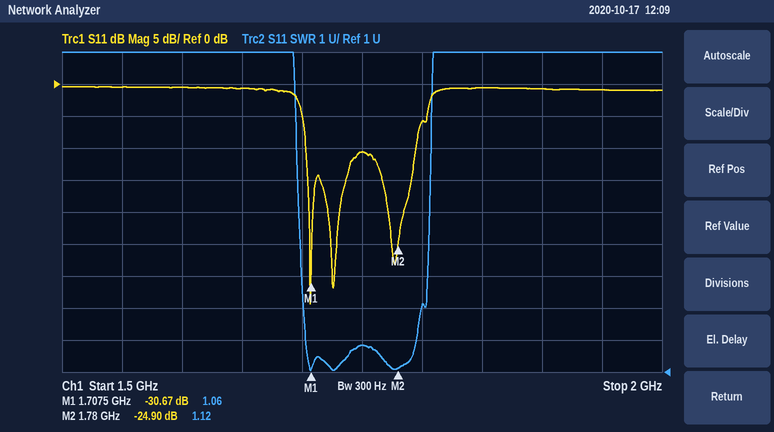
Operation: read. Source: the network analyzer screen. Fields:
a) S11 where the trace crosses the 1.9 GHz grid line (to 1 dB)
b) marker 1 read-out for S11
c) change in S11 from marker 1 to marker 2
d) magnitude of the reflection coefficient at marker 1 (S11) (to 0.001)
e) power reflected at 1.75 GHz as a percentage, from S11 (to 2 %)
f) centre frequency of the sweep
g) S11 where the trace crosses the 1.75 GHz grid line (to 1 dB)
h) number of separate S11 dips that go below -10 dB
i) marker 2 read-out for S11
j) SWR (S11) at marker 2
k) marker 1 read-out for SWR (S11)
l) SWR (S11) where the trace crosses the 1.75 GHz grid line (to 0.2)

-1 dB
-30.67 dB
5.77 dB
0.029
8 %
1.75 GHz
-11 dB
3
-24.90 dB
1.12
1.06
1.8
